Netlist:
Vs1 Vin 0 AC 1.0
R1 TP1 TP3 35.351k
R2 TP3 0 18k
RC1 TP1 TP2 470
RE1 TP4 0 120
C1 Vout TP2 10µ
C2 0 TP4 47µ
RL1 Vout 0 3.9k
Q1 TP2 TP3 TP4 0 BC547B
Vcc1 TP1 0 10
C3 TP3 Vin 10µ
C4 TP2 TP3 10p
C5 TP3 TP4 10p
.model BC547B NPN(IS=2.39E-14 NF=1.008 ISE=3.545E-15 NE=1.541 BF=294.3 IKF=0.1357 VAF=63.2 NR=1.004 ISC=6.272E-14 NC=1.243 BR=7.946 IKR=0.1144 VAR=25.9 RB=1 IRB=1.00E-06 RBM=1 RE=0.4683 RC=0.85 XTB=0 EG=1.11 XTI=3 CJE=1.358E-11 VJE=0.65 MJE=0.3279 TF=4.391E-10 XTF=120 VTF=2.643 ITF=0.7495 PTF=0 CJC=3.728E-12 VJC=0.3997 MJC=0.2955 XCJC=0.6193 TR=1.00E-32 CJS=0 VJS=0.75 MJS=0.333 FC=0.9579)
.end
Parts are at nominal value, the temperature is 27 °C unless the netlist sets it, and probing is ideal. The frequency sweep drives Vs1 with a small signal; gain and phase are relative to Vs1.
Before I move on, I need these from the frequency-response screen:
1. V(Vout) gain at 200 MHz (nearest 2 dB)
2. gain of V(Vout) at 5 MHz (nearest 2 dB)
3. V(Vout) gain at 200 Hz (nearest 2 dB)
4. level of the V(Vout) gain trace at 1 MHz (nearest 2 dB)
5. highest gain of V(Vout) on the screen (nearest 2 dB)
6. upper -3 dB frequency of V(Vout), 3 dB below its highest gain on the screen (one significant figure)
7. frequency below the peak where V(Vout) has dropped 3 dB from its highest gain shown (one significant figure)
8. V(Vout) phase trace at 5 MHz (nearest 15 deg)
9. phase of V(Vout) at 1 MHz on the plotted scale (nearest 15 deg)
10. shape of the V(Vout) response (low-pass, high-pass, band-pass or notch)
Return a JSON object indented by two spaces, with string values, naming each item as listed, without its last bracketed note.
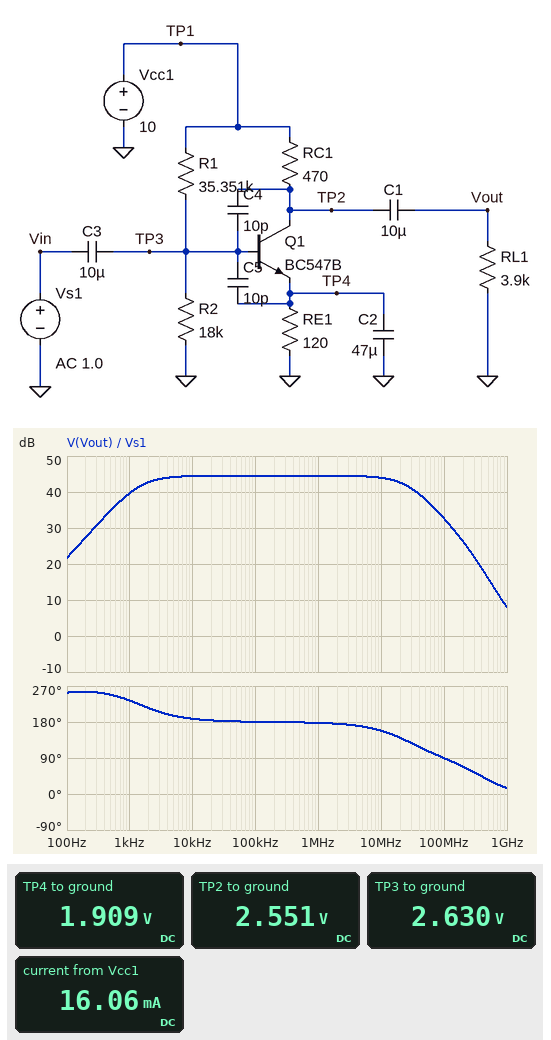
{
  "V(Vout) gain at 200 MHz": "26 dB",
  "gain of V(Vout) at 5 MHz": "44 dB",
  "V(Vout) gain at 200 Hz": "28 dB",
  "level of the V(Vout) gain trace at 1 MHz": "44 dB",
  "highest gain of V(Vout) on the screen": "44 dB",
  "upper -3 dB frequency of V(Vout), 3 dB below its highest gain on the screen": "30 MHz",
  "frequency below the peak where V(Vout) has dropped 3 dB from its highest gain shown": "1 kHz",
  "V(Vout) phase trace at 5 MHz": "165 deg",
  "phase of V(Vout) at 1 MHz on the plotted scale": "180 deg",
  "shape of the V(Vout) response": "band-pass"
}
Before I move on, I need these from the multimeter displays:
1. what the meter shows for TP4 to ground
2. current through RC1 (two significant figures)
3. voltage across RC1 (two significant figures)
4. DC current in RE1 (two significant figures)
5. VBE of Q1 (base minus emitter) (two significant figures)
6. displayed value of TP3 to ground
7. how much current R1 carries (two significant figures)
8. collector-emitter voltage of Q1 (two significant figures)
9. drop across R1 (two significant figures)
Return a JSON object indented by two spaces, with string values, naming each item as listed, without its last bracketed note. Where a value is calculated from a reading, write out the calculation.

{
  "what the meter shows for TP4 to ground": "1.909 V",
  "current through RC1": "(10 V - 2.551 V) / 470 Ω = 16 mA",
  "voltage across RC1": "10 V - 2.551 V = 7.4 V",
  "DC current in RE1": "(1.909 V) / 120 Ω = 16 mA",
  "VBE of Q1 (base minus emitter)": "2.63 V - 1.909 V = 720 mV",
  "displayed value of TP3 to ground": "2.630 V",
  "how much current R1 carries": "(10 V - 2.63 V) / 35.35 kΩ = 210 µA",
  "collector-emitter voltage of Q1": "2.551 V - 1.909 V = 640 mV",
  "drop across R1": "10 V - 2.63 V = 7.4 V"
}
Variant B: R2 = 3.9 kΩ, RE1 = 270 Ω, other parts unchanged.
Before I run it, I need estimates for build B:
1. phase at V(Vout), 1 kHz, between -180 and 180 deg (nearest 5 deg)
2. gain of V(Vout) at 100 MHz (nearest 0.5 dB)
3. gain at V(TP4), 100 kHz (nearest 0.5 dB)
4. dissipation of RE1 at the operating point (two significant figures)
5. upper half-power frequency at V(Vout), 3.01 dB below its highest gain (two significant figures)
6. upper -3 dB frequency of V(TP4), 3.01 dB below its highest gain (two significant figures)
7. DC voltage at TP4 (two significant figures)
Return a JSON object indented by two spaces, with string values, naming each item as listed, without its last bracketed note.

{
  "phase at V(Vout), 1 kHz, between -180 and 180 deg": "-170 deg",
  "gain of V(Vout) at 100 MHz": "16.0 dB",
  "gain at V(TP4), 100 kHz": "-56.0 dB",
  "dissipation of RE1 at the operating point": "420 µW",
  "upper half-power frequency at V(Vout), 3.01 dB below its highest gain": "33 MHz",
  "upper -3 dB frequency of V(TP4), 3.01 dB below its highest gain": "180 Hz",
  "DC voltage at TP4": "340 mV"
}
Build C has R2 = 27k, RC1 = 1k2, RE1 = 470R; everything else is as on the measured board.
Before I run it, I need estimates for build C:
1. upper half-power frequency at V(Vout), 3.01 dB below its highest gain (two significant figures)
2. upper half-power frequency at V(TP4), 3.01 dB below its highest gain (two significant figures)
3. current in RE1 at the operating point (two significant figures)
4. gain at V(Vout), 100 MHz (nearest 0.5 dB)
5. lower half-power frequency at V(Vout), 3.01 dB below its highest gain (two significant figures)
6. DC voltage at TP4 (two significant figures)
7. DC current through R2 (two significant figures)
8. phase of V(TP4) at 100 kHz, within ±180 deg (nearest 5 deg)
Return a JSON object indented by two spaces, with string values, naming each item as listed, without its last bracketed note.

{
  "upper half-power frequency at V(Vout), 3.01 dB below its highest gain": "25 MHz",
  "upper half-power frequency at V(TP4), 3.01 dB below its highest gain": "610 Hz",
  "current in RE1 at the operating point": "6.0 mA",
  "gain at V(Vout), 100 MHz": "14.0 dB",
  "lower half-power frequency at V(Vout), 3.01 dB below its highest gain": "590 Hz",
  "DC voltage at TP4": "2.8 V",
  "DC current through R2": "130 µA",
  "phase of V(TP4) at 100 kHz, within ±180 deg": "-90 deg"
}
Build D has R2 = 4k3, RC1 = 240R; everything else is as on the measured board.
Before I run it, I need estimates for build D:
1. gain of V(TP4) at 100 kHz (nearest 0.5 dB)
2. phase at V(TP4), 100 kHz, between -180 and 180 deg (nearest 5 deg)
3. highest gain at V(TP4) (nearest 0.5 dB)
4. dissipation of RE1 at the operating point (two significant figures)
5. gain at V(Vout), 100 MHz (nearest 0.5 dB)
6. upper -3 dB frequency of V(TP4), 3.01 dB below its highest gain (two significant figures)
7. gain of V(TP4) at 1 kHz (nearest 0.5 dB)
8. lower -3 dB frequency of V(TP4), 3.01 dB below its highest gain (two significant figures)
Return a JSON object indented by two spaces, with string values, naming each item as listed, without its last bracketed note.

{
  "gain of V(TP4) at 100 kHz": "-48.5 dB",
  "phase at V(TP4), 100 kHz, between -180 and 180 deg": "-90 deg",
  "highest gain at V(TP4)": "-1.0 dB",
  "dissipation of RE1 at the operating point": "1.2 mW",
  "gain at V(Vout), 100 MHz": "22.5 dB",
  "upper -3 dB frequency of V(TP4), 3.01 dB below its highest gain": "420 Hz",
  "gain of V(TP4) at 1 kHz": "-9.0 dB",
  "lower -3 dB frequency of V(TP4), 3.01 dB below its highest gain": "4.4 Hz"
}
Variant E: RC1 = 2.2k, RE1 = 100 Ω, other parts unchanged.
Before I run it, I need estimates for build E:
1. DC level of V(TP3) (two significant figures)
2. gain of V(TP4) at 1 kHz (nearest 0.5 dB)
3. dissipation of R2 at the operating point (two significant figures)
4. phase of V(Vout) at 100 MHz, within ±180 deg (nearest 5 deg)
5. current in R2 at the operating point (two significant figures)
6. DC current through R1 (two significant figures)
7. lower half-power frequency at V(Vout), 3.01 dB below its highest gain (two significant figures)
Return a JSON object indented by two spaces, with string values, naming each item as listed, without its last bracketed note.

{
  "DC level of V(TP3)": "1.1 V",
  "gain of V(TP4) at 1 kHz": "-21.5 dB",
  "dissipation of R2 at the operating point": "72 µW",
  "phase of V(Vout) at 100 MHz, within ±180 deg": "115 deg",
  "current in R2 at the operating point": "63 µA",
  "DC current through R1": "250 µA",
  "lower half-power frequency at V(Vout), 3.01 dB below its highest gain": "530 Hz"
}
